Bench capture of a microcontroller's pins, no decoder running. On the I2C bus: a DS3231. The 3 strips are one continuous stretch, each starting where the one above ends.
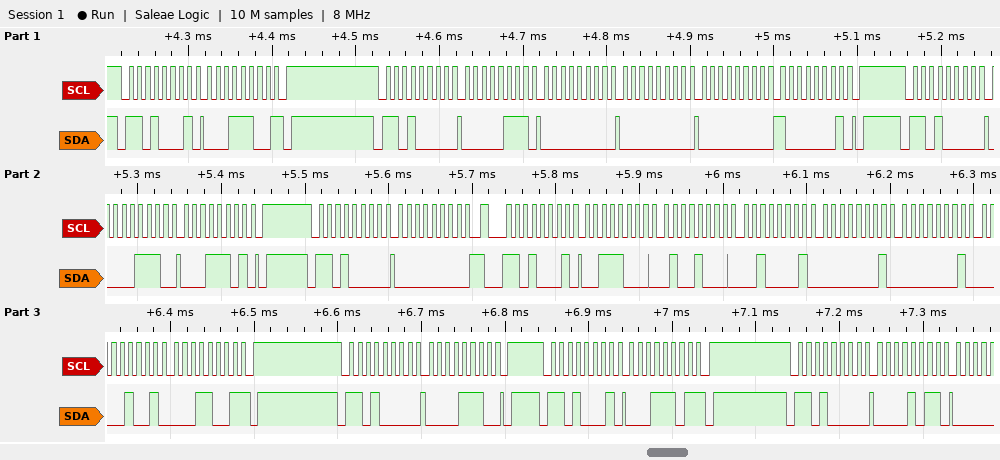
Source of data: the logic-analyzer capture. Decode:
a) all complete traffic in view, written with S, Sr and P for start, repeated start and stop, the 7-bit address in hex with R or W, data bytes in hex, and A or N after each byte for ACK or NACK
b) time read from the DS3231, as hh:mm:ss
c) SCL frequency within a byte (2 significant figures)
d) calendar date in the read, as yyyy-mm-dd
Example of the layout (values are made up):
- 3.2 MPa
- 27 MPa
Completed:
- S 68R A 1C N P S 68W A 07 A 00 A 00 A 00 A 81 A P S 68W A 0E A 1D A P S 68W A 00 A Sr 68R A 38 A 48 A 21 A 01 A 01 A 09 A 19 N P S 68W A 0E A P S 68R A 1D N P S 68W A 0B A
- 21:48:38
- 100 kHz
- 2019-09-01
